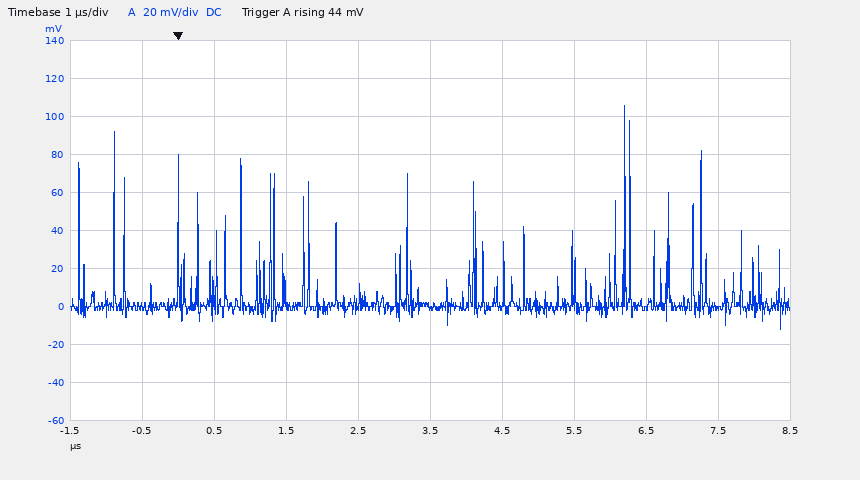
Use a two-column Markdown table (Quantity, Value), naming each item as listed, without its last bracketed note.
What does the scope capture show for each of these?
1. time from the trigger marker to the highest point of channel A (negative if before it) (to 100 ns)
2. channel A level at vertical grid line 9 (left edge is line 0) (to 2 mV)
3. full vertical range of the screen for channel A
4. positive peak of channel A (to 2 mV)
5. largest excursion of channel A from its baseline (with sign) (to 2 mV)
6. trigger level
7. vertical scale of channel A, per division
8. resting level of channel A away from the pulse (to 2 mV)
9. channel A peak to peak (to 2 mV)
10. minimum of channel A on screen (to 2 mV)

| Quantity | Value |
|---|---|
| time from the trigger marker to the highest point of channel A (negative if before it) | +6.2 µs |
| channel A level at vertical grid line 9 (left edge is line 0) | 0 mV |
| full vertical range of the screen for channel A | 200 mV |
| positive peak of channel A | 106 mV |
| largest excursion of channel A from its baseline (with sign) | +106 mV |
| trigger level | 44 mV |
| vertical scale of channel A, per division | 20 mV |
| resting level of channel A away from the pulse | 0 mV |
| channel A peak to peak | 118 mV |
| minimum of channel A on screen | -12 mV |
